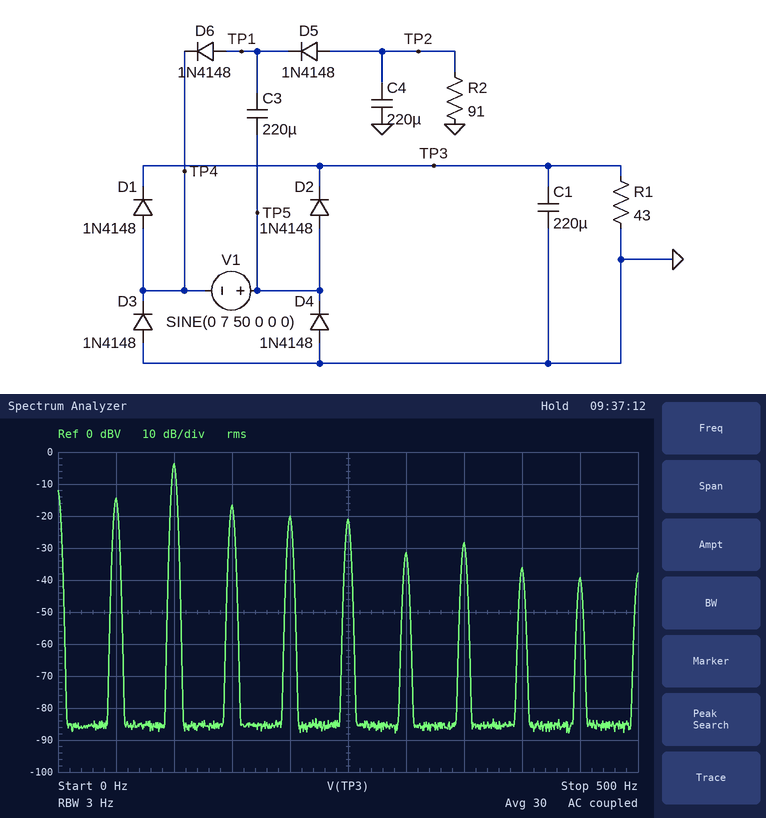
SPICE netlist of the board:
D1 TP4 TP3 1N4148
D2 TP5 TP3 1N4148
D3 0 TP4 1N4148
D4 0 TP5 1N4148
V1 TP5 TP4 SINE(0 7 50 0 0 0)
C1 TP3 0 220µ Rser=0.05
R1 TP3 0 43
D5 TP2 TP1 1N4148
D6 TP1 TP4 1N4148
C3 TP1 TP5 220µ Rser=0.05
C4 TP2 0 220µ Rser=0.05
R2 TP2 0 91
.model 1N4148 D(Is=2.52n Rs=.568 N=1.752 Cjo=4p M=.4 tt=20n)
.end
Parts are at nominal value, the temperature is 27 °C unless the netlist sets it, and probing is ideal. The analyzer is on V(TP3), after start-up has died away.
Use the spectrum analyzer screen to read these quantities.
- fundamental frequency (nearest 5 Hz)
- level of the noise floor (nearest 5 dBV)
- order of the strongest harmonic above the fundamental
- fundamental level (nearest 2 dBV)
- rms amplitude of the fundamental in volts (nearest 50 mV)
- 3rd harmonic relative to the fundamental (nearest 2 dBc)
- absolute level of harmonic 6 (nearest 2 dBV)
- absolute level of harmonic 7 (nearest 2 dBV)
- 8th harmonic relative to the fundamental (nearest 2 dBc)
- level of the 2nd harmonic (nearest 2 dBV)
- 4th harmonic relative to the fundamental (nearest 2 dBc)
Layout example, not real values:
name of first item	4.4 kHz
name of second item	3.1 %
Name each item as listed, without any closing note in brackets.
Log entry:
fundamental frequency	50 Hz
level of the noise floor	-85 dBV
order of the strongest harmonic above the fundamental	2
fundamental level	-14 dBV
rms amplitude of the fundamental in volts	200 mV
3rd harmonic relative to the fundamental	-2 dBc
absolute level of harmonic 6	-32 dBV
absolute level of harmonic 7	-28 dBV
8th harmonic relative to the fundamental	-22 dBc
level of the 2nd harmonic	-4 dBV
4th harmonic relative to the fundamental	-6 dBc
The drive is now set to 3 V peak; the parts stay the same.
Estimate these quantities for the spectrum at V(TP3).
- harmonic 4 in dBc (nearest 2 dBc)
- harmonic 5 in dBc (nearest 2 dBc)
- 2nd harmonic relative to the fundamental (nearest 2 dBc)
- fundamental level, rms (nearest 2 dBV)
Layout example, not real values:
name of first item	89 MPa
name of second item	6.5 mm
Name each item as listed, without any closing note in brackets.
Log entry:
harmonic 4 in dBc	-8 dBc
harmonic 5 in dBc	-8 dBc
2nd harmonic relative to the fundamental	8 dBc
fundamental level, rms	-22 dBV
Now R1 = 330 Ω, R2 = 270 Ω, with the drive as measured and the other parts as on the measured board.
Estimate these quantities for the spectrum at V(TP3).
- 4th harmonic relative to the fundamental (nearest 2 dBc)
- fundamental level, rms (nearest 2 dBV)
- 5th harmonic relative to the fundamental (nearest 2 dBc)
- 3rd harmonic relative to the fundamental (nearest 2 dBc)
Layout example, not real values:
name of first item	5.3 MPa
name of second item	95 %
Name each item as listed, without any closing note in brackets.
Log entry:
4th harmonic relative to the fundamental	-18 dBc
fundamental level, rms	-12 dBV
5th harmonic relative to the fundamental	-18 dBc
3rd harmonic relative to the fundamental	-10 dBc
